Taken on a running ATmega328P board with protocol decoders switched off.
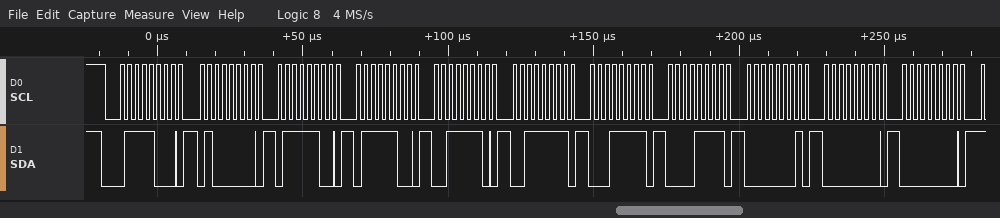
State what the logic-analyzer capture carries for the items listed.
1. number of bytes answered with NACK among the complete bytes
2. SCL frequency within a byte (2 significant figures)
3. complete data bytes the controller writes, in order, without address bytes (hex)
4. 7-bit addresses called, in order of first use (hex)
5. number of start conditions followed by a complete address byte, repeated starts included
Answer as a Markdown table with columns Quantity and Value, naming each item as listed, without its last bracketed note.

| Quantity | Value |
|---|---|
| number of bytes answered with NACK among the complete bytes | 0 |
| SCL frequency within a byte | 400 kHz |
| complete data bytes the controller writes, in order, without address bytes | 40 7C 7C 3E 3F 1F 0F 01 00 00 |
| 7-bit addresses called, in order of first use | 0x3C |
| number of start conditions followed by a complete address byte, repeated starts included | 1 |
